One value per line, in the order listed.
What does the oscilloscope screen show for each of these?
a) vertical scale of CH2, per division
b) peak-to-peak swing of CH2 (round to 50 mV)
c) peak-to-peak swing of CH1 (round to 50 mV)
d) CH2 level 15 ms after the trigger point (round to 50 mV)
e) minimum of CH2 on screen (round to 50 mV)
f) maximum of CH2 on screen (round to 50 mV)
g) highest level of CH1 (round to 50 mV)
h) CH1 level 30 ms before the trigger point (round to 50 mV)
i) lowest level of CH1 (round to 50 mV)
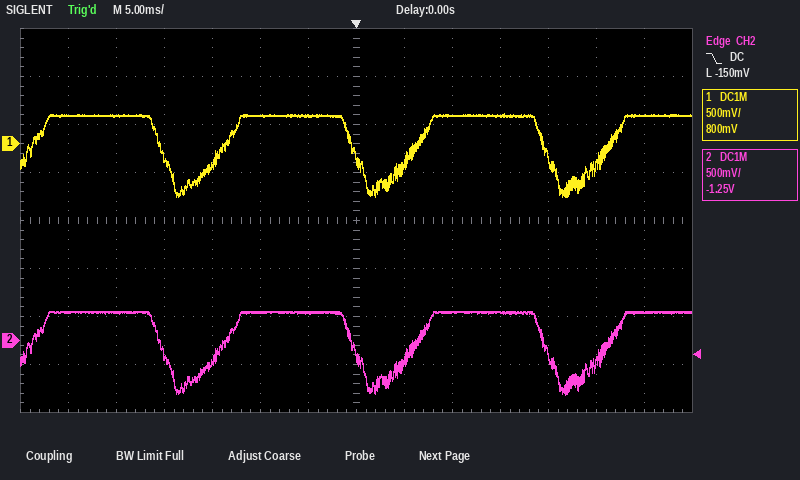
500 mV
850 mV
850 mV
300 mV
-550 mV
300 mV
300 mV
300 mV
-550 mV
